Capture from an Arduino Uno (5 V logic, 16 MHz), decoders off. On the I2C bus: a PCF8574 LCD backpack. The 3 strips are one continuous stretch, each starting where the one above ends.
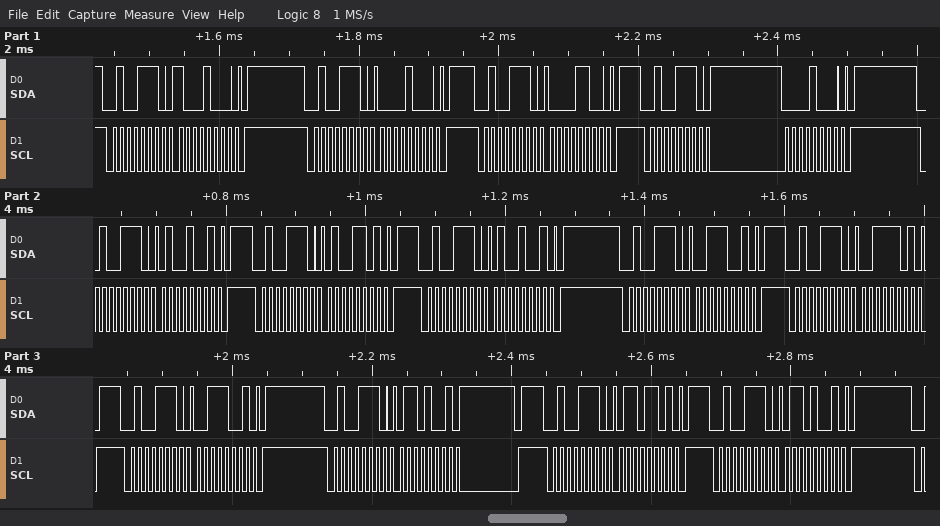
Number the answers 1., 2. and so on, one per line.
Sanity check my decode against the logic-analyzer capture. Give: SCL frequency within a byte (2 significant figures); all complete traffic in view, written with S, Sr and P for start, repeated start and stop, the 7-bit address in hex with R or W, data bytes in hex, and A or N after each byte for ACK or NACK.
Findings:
1. 100 kHz
2. S 27W A 88 A P S 27W A 08 A P S 27W A 0C A P S 27W A 08 A P S 27W A 49 A P S 27W A 4D A P S 27W A 49 A P S 27W A 39 A P S 27W A 3D A P S 27W A 39 A P S 27W A 69 A P S 27W A 6D A P S 27W A 69 A P
